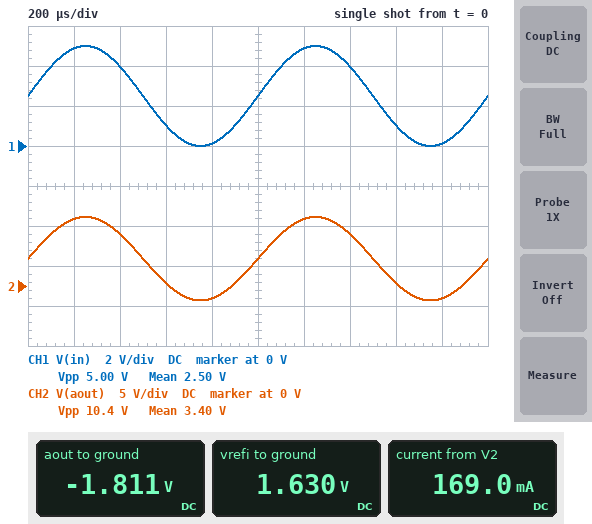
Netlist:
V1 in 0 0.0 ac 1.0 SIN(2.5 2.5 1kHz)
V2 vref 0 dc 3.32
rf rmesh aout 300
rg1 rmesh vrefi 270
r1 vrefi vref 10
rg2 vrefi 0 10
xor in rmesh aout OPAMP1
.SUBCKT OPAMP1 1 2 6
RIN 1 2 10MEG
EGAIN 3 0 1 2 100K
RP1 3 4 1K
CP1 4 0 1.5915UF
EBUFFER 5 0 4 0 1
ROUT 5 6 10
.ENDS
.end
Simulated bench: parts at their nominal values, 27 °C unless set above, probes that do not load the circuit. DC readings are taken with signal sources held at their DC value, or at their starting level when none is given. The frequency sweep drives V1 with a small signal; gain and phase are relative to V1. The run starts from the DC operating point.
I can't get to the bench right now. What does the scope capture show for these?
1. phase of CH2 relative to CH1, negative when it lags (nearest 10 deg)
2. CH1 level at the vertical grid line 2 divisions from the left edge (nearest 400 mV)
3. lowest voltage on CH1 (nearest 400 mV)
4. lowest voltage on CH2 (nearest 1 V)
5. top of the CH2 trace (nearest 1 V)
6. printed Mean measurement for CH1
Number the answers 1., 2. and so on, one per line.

1. 0 deg
2. 4.0 V
3. 0 V
4. -2 V
5. 9 V
6. 2.50 V
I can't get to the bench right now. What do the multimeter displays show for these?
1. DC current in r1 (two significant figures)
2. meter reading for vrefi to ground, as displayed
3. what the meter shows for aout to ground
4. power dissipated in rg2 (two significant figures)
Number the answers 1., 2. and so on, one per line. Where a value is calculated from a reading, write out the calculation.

1. (3.32 V - 1.63 V) / 10 Ω = 170 mA
2. 1.630 V
3. -1.811 V
4. (1.63 V)^2 / 10 Ω = 270 mW
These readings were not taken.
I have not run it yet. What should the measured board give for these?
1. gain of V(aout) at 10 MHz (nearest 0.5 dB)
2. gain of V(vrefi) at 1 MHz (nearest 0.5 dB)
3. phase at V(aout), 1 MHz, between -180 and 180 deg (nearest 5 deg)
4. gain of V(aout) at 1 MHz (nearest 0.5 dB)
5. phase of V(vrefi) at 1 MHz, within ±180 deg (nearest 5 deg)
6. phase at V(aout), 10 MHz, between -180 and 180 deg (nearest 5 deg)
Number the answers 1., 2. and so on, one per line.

1. -1.0 dB
2. -35.0 dB
3. -10 deg
4. 6.0 dB
5. -10 deg
6. -65 deg
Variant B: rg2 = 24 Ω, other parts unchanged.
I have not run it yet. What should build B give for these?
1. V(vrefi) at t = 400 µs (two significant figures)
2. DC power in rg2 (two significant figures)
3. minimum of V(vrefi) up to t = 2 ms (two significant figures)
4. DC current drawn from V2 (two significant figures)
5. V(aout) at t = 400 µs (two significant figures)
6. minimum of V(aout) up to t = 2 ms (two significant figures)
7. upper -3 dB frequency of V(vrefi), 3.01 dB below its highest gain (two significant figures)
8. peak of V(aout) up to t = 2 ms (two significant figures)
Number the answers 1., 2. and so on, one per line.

1. 2.4 V
2. 220 mW
3. 2.3 V
4. 100 mA
5. 5.7 V
6. -2.5 V
7. 4.7 MHz
8. 7.9 V
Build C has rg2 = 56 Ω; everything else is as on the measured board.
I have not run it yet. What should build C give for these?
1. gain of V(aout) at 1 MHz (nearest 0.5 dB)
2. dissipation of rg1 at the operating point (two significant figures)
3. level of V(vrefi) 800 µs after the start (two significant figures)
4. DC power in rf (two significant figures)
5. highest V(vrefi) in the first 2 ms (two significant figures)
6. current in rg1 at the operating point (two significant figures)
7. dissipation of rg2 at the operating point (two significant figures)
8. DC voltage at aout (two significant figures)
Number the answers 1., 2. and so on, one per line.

1. 6.0 dB
2. 28 mW
3. 2.7 V
4. 31 mW
5. 2.9 V
6. 10 mA
7. 130 mW
8. -3.0 V
